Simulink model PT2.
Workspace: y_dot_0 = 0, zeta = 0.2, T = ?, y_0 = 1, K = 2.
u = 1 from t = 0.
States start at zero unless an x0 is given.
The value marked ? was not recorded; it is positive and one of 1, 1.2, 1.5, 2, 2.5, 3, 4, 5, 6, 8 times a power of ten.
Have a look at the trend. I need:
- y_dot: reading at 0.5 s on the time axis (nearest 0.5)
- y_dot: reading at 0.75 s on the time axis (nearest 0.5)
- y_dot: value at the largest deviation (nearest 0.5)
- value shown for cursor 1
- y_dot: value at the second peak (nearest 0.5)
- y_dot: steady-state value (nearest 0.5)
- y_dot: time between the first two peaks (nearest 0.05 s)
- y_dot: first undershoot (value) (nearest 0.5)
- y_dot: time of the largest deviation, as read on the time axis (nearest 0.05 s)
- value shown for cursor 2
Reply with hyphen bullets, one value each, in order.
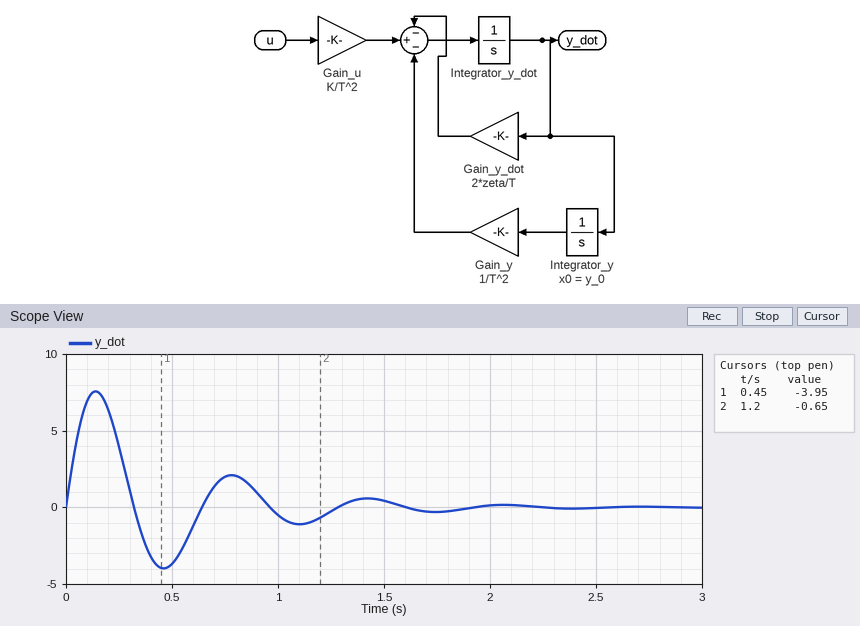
- -3.5
- 2.0
- 7.5
- -3.95
- 2.0
- 0.0
- 0.65 s
- -4.0
- 0.15 s
- -0.65
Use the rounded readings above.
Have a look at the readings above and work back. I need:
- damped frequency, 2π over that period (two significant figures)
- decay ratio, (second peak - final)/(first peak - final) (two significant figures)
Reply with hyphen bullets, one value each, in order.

- 9.7 rad/s
- 0.27
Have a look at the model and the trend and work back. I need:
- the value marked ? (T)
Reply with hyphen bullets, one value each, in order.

- 0.1
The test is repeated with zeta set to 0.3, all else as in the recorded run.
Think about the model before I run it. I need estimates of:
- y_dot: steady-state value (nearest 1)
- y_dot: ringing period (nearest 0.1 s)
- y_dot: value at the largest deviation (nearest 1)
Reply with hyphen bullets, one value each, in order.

- 0
- 0.7 s
- 7
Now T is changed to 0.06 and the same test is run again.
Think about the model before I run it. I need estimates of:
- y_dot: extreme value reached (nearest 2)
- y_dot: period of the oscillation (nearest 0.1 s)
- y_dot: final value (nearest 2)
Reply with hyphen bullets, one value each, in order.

- 12
- 0.4 s
- 0
